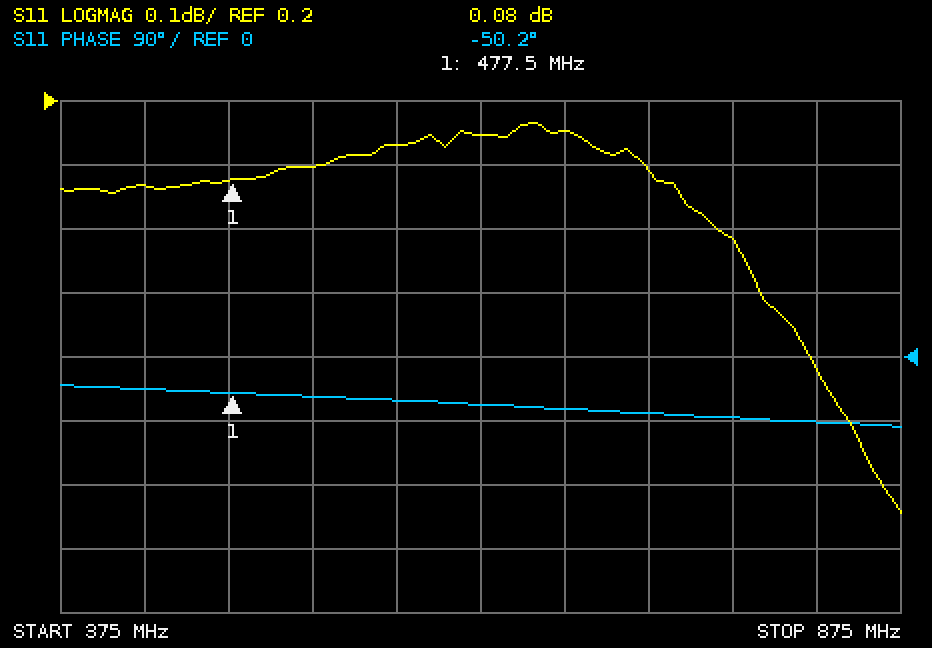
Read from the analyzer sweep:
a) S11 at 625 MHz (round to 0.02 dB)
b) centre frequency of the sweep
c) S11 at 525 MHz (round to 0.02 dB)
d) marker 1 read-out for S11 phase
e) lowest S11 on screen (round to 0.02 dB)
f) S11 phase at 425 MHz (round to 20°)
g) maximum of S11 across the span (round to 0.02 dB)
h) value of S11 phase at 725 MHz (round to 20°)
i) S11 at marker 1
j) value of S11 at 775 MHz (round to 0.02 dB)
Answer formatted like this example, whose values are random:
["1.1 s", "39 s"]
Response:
["0.14 dB", "625 MHz", "0.10 dB", "-50.2°", "-0.44 dB", "-40°", "0.16 dB", "-80°", "0.08 dB", "-0.02 dB"]
